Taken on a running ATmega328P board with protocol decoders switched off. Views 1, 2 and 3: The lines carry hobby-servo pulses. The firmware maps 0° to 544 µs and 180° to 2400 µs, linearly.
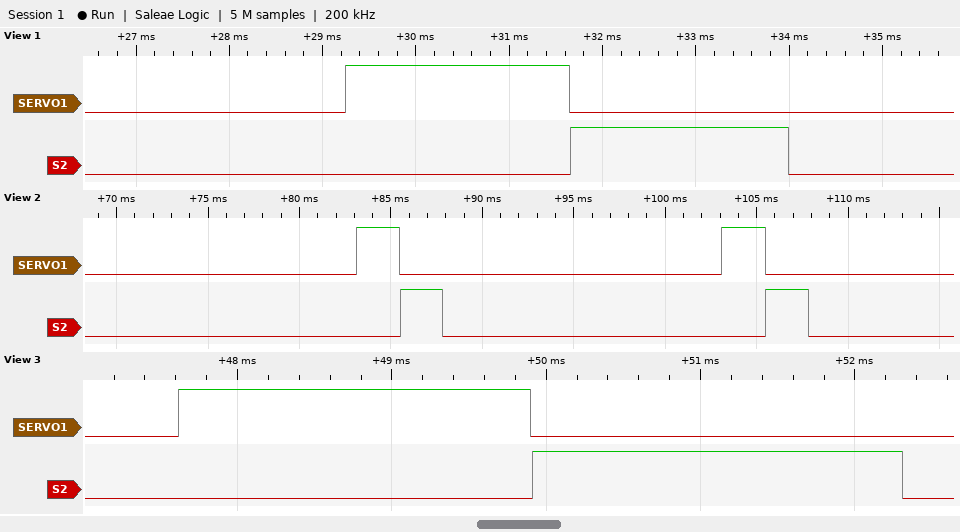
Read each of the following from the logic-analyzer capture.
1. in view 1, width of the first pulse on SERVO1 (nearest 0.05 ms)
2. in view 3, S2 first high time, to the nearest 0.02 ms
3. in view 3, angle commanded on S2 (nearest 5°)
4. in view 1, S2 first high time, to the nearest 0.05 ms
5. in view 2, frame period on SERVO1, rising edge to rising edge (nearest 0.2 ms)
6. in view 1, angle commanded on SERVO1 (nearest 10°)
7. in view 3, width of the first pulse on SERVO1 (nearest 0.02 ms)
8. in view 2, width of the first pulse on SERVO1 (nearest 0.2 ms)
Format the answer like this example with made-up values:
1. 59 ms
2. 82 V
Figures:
1. 2.40 ms
2. 2.40 ms
3. 180°
4. 2.35 ms
5. 20.0 ms
6. 180°
7. 2.28 ms
8. 2.4 ms
